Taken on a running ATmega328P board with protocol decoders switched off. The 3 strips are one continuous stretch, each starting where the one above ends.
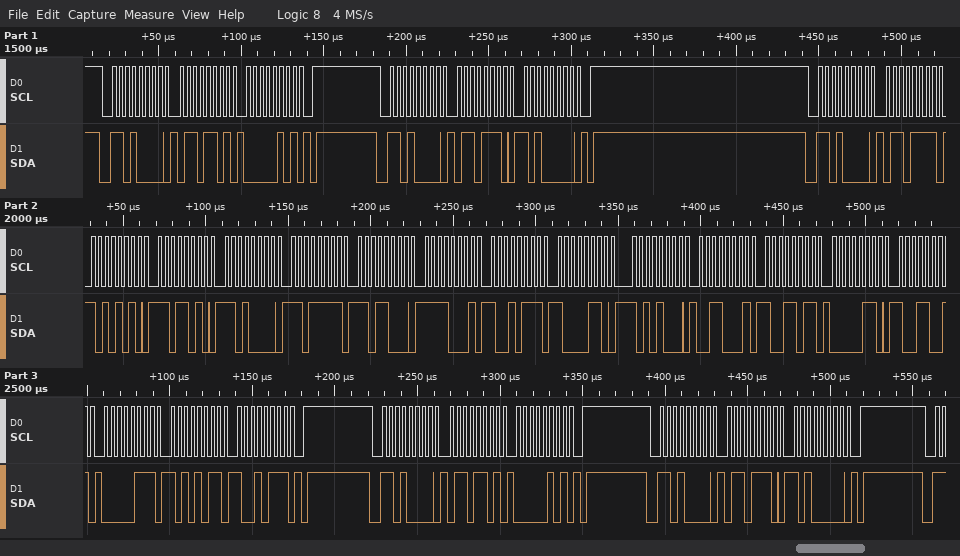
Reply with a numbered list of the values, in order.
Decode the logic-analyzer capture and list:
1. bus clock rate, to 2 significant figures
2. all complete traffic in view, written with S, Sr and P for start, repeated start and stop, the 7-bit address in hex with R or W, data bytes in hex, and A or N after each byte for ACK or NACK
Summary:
1. 250 kHz
2. S 68W A 6D A 05 A P S 68W A 6E A A0 A P S 68W A 6F A AA A DA A D0 A DF A D8 A F1 A 97 A 86 A A8 A 31 A 9B A 06 A 99 A 07 A AB A 97 A P S 68W A 6D A 05 A P S 68W A 6E A A0 A P
